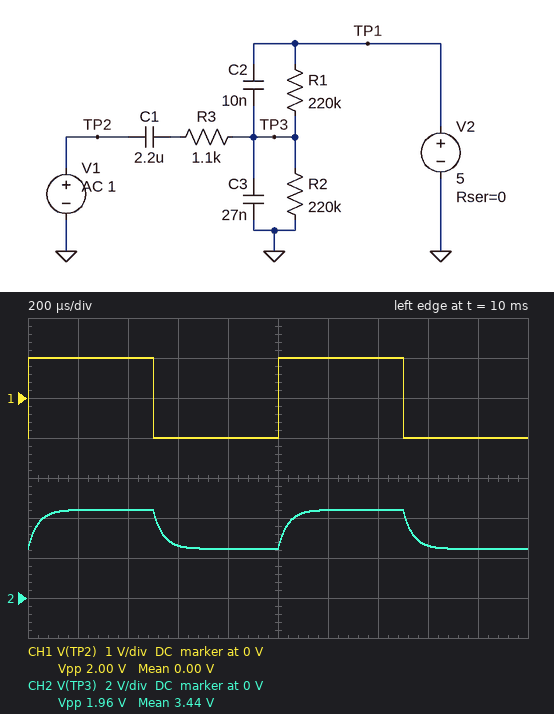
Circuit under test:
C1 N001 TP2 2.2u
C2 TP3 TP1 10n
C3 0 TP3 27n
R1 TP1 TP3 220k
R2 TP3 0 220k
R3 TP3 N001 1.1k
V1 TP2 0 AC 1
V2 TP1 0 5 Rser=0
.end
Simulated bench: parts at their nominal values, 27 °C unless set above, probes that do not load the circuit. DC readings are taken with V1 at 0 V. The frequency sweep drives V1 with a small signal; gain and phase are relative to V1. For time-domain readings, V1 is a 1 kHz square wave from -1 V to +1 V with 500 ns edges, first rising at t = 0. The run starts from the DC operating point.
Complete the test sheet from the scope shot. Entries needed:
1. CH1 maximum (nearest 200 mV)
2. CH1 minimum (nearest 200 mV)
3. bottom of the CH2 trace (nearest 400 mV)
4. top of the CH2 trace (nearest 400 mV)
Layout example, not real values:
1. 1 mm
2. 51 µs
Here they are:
1. 1.0 V
2. -1.0 V
3. 2.4 V
4. 4.4 V
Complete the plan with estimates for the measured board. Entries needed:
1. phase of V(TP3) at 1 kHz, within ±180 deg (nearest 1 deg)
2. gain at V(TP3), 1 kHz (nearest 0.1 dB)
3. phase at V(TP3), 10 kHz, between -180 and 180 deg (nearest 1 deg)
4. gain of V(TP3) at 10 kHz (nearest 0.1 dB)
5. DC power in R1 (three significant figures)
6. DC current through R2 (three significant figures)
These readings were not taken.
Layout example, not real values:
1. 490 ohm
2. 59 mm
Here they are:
1. -14 deg
2. -0.5 dB
3. -68 deg
4. -8.8 dB
5. 28.4 µW
6. 11.4 µA
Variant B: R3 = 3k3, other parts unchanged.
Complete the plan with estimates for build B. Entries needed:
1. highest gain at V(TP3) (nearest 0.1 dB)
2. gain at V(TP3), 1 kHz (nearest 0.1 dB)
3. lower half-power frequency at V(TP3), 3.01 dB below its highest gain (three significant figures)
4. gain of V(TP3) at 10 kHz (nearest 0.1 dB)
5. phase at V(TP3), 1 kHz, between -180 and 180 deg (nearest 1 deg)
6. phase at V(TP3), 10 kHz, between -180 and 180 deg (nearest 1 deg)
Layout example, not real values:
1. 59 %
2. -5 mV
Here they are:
1. -0.4 dB
2. -2.3 dB
3. 628 mHz
4. -17.8 dB
5. -36 deg
6. -82 deg
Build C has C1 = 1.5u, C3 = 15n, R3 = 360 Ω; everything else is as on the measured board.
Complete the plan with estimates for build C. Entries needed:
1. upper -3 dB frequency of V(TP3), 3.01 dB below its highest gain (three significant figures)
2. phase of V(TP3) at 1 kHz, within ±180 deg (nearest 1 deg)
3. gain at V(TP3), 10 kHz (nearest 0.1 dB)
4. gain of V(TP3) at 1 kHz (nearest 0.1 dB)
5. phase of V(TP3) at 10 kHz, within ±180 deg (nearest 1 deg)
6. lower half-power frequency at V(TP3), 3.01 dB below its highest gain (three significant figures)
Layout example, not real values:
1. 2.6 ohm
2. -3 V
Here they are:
1. 18.0 kHz
2. -3 deg
3. -1.3 dB
4. -0.2 dB
5. -29 deg
6. 946 mHz
